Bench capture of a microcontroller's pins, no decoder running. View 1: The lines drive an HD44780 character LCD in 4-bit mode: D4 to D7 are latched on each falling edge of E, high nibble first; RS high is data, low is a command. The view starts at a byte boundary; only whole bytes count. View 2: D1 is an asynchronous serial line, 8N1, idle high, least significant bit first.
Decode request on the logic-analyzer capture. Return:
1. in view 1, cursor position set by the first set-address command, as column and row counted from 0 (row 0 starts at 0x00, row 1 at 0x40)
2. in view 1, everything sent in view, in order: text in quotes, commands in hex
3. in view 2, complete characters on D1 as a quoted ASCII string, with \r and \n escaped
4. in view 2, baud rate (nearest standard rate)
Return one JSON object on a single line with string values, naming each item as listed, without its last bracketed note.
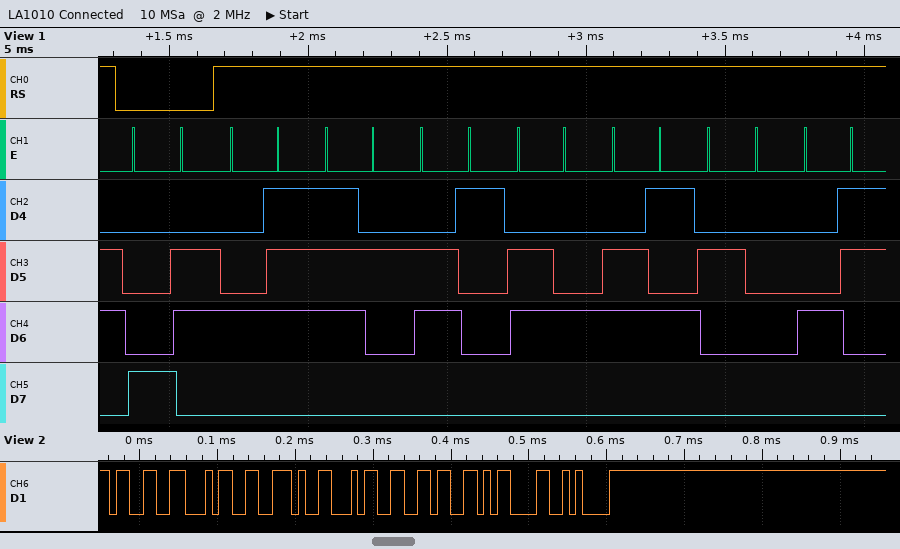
{"in view 1, cursor position set by the first set-address command, as column and row counted from 0": "column 6, row 0", "in view 1, everything sent in view, in order: text in quotes, commands in hex": "0x86 \"Grade C\"", "in view 2, complete characters on D1 as a quoted ASCII string, with \\r and \\n escaped": "\"34.46\\r\\n\"", "in view 2, baud rate": "115200 baud"}
